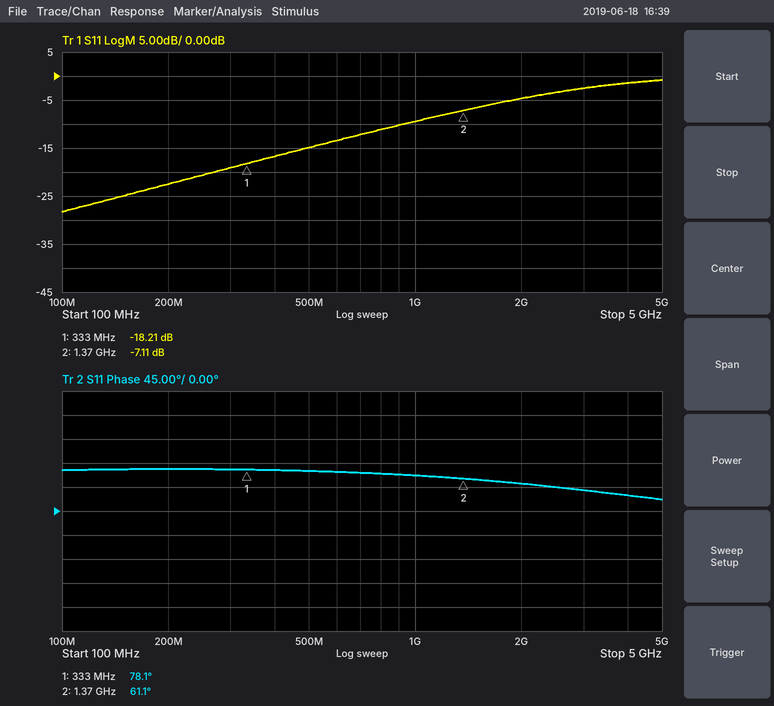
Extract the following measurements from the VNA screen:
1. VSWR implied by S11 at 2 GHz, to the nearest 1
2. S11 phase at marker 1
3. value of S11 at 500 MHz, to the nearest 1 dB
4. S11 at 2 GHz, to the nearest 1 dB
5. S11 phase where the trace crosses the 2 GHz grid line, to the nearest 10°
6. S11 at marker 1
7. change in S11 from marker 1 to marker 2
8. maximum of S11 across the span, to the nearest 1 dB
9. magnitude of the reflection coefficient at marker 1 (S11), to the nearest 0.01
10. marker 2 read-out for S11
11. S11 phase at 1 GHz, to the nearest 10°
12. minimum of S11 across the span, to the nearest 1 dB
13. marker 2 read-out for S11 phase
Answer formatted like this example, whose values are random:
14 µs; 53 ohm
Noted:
4; 78.1°; -15 dB; -5 dB; 50°; -18.21 dB; 11.10 dB; -1 dB; 0.12; -7.11 dB; 70°; -28 dB; 61.1°
